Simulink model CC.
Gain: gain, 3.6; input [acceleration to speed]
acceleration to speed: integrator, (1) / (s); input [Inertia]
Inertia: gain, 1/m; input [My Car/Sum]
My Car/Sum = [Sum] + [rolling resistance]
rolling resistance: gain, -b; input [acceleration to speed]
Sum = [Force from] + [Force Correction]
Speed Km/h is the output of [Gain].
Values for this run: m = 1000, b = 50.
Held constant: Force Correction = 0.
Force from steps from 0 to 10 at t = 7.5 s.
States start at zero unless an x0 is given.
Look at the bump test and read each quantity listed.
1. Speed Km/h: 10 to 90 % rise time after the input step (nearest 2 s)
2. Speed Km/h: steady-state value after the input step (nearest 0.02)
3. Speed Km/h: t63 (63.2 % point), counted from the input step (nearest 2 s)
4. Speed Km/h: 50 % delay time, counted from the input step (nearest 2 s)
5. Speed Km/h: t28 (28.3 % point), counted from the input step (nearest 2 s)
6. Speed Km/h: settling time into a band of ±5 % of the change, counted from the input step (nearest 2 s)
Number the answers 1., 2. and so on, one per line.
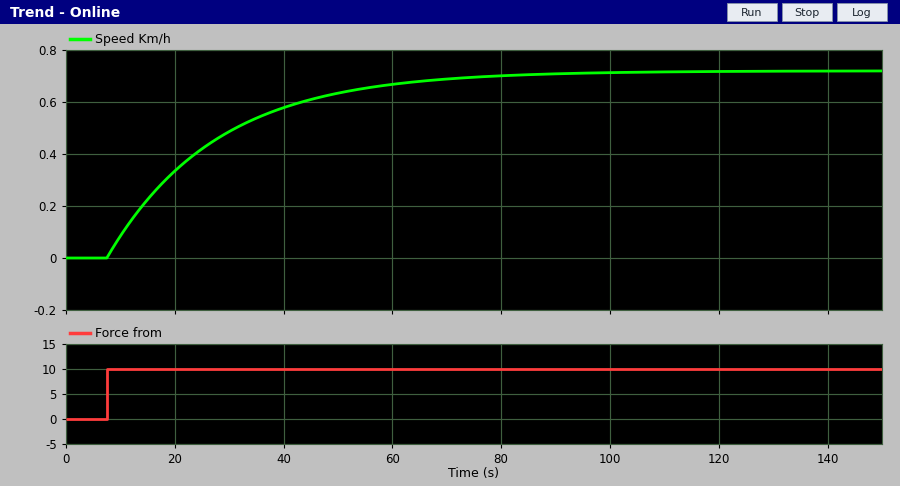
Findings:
1. 44 s
2. 0.72
3. 20 s
4. 14 s
5. 6 s
6. 60 s
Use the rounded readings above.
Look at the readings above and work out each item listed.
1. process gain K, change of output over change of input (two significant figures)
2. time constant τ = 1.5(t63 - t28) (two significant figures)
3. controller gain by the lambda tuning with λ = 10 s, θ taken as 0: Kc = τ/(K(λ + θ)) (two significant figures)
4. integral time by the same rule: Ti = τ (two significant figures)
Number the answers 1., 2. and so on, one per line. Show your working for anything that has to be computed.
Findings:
1. (0.72 - 0) / 10 = 0.072
2. 1.5 × (20 - 6) = 21 s
3. 21 / (0.072 × (10 + 0)) = 29
4. 21 s
